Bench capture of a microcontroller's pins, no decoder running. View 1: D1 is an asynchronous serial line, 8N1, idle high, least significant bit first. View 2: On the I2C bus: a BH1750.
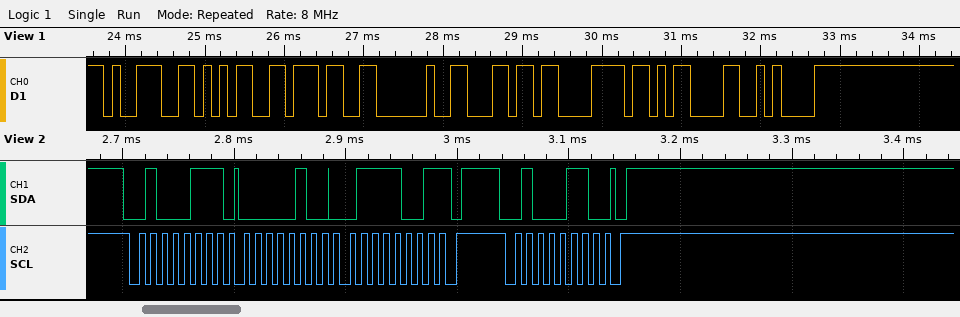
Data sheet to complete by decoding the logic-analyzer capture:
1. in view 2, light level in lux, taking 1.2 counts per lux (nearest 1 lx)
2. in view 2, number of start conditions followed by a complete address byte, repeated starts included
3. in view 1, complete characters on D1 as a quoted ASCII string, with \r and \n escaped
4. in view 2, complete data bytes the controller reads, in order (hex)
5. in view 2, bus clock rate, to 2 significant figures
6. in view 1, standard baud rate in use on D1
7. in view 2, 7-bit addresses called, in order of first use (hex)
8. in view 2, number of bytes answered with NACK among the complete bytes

954 lx
2
"957 lx\r\n"
04 79
100 kHz
9600 baud
0x23
1
